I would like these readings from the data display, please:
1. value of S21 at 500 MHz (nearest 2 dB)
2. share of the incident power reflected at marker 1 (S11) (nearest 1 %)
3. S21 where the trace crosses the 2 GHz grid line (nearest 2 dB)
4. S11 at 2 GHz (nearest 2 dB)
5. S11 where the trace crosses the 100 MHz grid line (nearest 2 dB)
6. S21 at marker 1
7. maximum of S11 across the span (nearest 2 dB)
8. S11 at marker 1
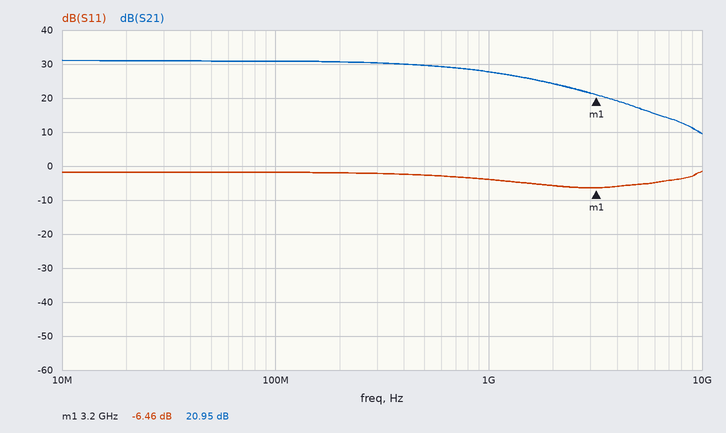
30 dB
23 %
24 dB
-6 dB
-2 dB
20.95 dB
-2 dB
-6.46 dB
